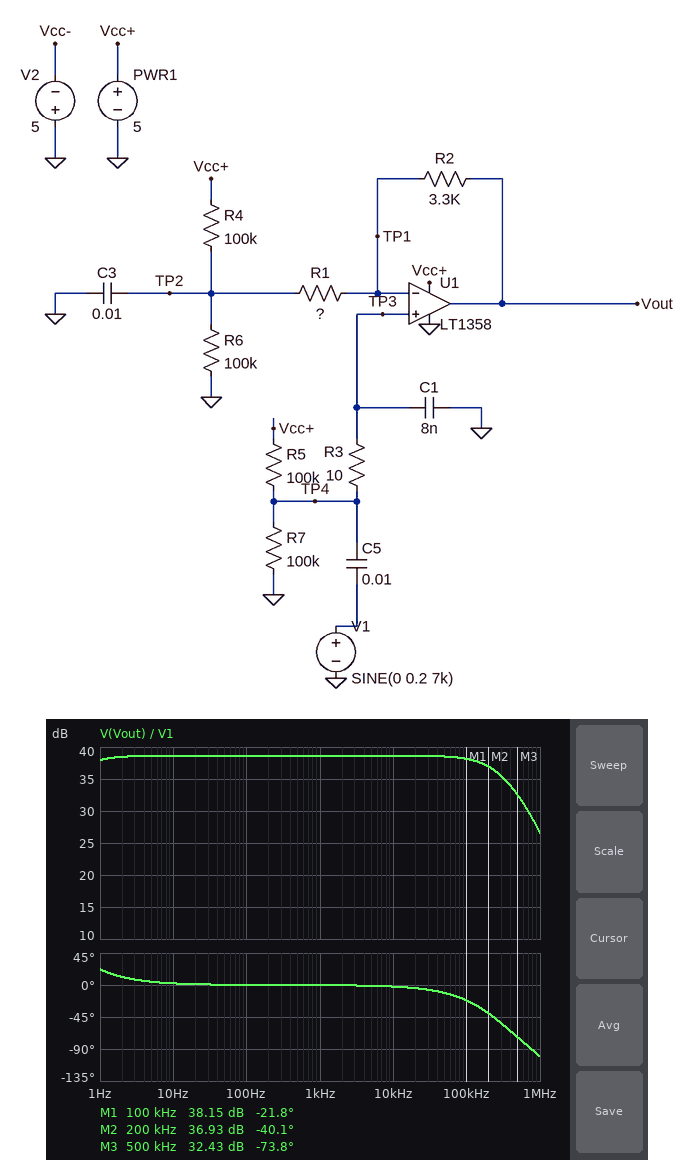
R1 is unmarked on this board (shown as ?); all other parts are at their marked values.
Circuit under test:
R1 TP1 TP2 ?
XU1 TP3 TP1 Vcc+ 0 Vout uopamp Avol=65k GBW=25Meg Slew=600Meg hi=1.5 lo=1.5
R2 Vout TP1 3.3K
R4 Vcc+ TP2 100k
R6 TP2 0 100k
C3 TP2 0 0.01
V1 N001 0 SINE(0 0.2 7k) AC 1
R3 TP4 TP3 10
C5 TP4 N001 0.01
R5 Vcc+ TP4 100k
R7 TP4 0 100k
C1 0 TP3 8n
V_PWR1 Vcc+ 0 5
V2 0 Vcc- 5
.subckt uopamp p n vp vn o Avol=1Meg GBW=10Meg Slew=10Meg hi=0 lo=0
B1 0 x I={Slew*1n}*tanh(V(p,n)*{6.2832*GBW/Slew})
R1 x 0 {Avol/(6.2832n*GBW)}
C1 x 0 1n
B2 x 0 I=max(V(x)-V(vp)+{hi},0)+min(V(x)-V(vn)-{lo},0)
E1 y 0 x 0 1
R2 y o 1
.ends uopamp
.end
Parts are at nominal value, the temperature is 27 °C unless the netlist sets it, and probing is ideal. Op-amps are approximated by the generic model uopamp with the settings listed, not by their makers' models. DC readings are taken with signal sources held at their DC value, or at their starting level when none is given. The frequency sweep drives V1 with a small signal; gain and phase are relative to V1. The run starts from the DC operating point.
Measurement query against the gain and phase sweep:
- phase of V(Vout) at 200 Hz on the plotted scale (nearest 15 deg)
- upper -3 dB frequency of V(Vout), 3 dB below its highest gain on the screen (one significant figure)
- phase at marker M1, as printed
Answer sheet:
0 deg
300 kHz
-21.8 deg
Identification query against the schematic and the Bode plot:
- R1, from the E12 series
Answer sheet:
39 Ω
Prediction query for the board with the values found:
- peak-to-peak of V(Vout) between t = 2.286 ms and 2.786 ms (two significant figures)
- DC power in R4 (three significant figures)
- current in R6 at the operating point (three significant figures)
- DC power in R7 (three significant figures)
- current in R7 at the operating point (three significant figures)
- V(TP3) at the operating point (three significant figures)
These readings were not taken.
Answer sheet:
2.1 V
62.5 µW
25.0 µA
62.5 µW
25.0 µA
2.50 V
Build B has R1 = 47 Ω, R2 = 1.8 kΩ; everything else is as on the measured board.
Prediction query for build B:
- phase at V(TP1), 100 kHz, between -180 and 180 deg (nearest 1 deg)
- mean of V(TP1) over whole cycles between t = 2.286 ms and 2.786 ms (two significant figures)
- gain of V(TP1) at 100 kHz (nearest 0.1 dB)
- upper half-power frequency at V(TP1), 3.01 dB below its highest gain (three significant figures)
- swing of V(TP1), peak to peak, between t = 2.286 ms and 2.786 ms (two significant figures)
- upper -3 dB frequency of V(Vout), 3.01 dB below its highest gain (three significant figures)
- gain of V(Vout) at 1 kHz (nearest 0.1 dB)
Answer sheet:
-12 deg
2.5 V
-0.1 dB
583 kHz
52 mV
584 kHz
31.9 dB
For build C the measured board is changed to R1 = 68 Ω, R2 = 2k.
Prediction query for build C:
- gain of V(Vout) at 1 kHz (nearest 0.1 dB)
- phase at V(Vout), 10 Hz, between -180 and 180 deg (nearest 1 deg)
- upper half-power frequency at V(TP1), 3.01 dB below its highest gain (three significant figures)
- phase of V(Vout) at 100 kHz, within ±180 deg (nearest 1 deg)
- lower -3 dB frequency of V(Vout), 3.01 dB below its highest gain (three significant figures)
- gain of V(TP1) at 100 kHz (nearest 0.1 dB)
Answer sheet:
29.7 dB
1 deg
720 kHz
-10 deg
234 mHz
-0.1 dB
